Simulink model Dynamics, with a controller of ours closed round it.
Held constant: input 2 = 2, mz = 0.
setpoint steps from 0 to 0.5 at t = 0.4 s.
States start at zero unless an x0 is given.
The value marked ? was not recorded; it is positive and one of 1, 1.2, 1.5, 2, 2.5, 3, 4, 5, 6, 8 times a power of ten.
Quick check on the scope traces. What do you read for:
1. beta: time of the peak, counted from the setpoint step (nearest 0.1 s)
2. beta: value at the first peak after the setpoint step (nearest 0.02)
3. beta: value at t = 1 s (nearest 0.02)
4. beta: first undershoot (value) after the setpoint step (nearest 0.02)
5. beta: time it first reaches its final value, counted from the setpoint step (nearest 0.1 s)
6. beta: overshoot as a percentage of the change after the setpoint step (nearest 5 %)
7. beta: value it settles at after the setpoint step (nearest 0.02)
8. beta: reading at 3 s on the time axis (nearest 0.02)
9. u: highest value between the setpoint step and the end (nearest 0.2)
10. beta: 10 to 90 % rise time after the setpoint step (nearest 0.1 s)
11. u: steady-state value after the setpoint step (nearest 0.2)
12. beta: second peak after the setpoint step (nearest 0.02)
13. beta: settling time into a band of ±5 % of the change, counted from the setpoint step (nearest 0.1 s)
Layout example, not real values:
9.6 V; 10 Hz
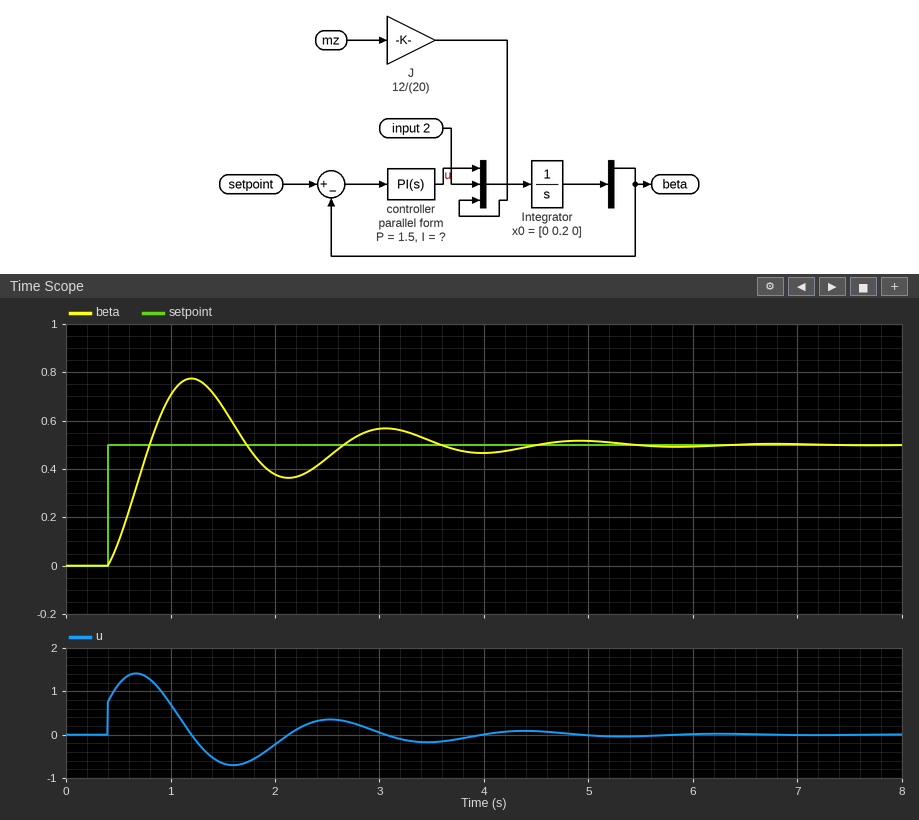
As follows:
0.8 s; 0.78; 0.70; 0.36; 0.4 s; 55 %; 0.50; 0.56; 1.4; 0.3 s; 0.0; 0.56; 3.8 s
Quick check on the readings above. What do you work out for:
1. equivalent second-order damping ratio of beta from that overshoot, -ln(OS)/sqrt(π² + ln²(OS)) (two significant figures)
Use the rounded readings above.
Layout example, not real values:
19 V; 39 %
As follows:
0.19
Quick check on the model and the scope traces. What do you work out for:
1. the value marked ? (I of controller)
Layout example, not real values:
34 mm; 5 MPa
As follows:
12
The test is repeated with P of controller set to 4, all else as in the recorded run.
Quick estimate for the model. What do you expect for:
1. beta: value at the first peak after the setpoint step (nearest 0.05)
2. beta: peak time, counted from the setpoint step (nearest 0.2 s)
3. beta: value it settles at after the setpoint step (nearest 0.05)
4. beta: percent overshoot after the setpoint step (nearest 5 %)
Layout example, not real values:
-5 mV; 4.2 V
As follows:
0.65; 0.6 s; 0.50; 25 %
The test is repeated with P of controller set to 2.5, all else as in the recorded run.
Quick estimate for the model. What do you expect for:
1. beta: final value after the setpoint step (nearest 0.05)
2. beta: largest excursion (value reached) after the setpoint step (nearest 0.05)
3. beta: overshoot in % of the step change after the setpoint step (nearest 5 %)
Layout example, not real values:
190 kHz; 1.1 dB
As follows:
0.50; 0.70; 40 %
